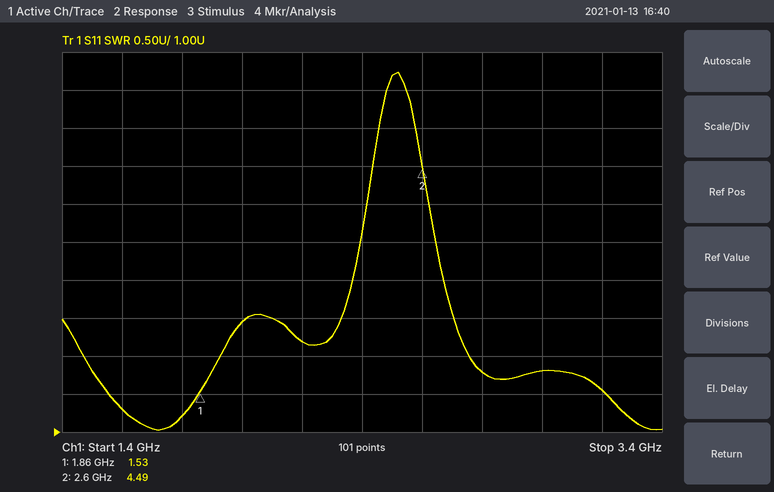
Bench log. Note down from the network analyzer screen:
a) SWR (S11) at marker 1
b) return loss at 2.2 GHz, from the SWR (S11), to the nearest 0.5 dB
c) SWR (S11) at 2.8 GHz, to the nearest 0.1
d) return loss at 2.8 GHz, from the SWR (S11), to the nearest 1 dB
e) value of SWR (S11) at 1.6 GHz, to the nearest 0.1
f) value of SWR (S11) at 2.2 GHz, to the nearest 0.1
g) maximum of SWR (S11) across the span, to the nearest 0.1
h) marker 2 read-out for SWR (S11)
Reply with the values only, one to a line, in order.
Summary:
1.53
8.5 dB
1.8
11 dB
1.3
2.2
5.7
4.49
